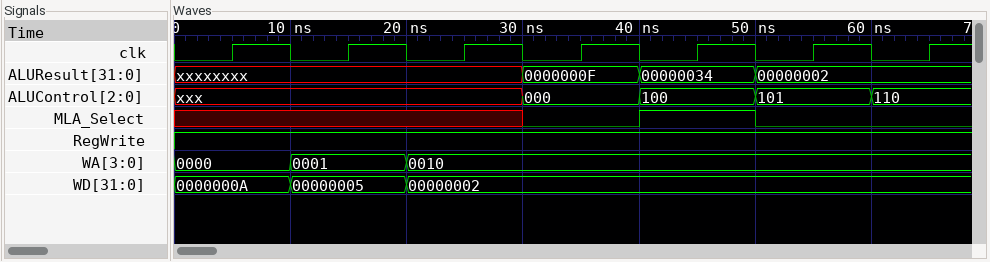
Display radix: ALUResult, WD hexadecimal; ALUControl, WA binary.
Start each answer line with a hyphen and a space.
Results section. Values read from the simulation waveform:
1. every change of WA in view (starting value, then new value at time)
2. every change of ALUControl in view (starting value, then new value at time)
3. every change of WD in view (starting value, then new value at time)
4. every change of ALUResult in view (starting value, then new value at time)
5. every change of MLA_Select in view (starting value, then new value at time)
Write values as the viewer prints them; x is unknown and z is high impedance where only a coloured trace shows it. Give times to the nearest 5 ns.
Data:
- 0000, 0001 at 10 ns, 0010 at 20 ns
- xxx, 000 at 30 ns, 100 at 40 ns, 101 at 50 ns, 110 at 60 ns
- 0000000A, 00000005 at 10 ns, 00000002 at 20 ns
- xxxxxxxx, 0000000F at 30 ns, 00000034 at 40 ns, 00000002 at 50 ns
- x, 0 at 30 ns, 1 at 40 ns, 0 at 50 ns
